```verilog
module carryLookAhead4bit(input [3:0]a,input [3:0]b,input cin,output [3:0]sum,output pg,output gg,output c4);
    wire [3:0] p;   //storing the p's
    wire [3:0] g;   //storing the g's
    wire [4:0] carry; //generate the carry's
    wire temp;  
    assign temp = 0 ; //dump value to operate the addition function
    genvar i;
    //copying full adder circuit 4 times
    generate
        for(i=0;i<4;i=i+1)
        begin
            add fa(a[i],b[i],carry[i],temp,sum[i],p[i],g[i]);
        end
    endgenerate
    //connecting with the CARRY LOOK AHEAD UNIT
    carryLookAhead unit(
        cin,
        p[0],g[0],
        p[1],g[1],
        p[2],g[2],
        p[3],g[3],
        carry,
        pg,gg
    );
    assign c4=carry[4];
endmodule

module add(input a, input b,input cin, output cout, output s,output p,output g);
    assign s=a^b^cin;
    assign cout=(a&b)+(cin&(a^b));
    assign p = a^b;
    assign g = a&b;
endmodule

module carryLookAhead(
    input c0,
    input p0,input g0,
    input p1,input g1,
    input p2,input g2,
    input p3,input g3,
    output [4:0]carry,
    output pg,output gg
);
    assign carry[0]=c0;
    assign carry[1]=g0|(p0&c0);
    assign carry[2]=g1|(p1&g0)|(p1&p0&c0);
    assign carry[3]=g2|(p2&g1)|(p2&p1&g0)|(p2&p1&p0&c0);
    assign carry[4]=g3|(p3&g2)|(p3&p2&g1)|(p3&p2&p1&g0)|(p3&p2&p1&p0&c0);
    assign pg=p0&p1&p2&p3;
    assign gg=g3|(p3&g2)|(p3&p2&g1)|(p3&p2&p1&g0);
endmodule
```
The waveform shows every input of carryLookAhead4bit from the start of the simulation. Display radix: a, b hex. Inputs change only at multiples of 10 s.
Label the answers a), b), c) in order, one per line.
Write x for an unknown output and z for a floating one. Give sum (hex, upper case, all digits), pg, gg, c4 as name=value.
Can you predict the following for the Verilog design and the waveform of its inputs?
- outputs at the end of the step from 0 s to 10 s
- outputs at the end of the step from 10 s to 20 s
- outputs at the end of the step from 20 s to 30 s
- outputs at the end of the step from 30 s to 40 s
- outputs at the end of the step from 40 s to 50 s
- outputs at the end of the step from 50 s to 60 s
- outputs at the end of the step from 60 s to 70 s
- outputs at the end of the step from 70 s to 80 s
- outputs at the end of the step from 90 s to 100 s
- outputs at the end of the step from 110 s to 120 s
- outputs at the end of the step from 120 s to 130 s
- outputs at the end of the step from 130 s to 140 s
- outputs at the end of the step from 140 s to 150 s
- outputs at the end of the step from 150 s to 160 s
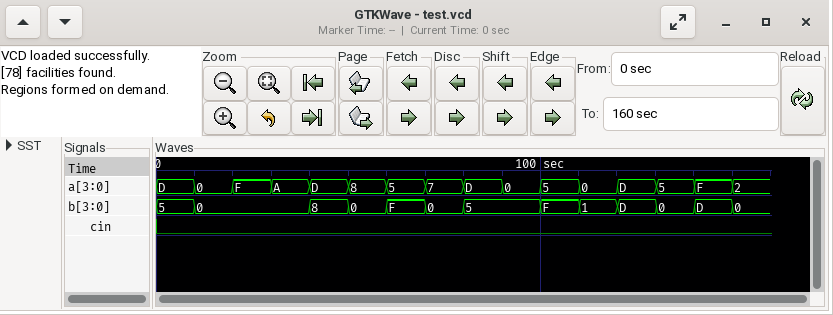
a) sum=2, pg=0, gg=1, c4=1
b) sum=0, pg=0, gg=0, c4=0
c) sum=F, pg=1, gg=0, c4=0
d) sum=A, pg=0, gg=0, c4=0
e) sum=5, pg=0, gg=1, c4=1
f) sum=8, pg=0, gg=0, c4=0
g) sum=4, pg=0, gg=1, c4=1
h) sum=7, pg=0, gg=0, c4=0
i) sum=5, pg=0, gg=0, c4=0
j) sum=1, pg=0, gg=0, c4=0
k) sum=A, pg=0, gg=1, c4=1
l) sum=5, pg=0, gg=0, c4=0
m) sum=C, pg=0, gg=1, c4=1
n) sum=2, pg=0, gg=0, c4=0
